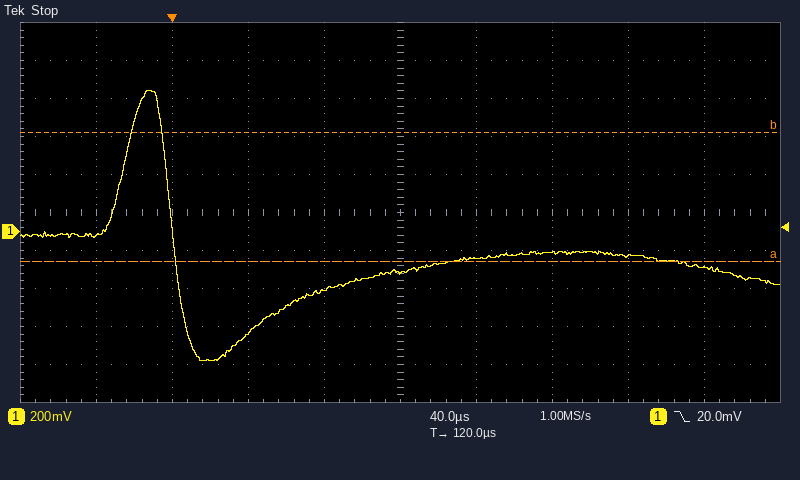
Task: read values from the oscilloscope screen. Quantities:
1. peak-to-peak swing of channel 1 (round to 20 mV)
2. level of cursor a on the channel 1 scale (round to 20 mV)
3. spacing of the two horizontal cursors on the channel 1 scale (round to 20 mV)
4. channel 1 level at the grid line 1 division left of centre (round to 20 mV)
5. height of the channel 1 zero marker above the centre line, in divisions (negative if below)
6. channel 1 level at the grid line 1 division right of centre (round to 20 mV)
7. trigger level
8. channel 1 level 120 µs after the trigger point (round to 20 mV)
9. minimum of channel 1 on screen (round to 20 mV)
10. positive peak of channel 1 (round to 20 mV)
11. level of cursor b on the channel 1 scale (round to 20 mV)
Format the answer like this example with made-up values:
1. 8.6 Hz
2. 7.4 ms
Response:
1. 1.42 V
2. -160 mV
3. 680 mV
4. -300 mV
5. -0.5 div
6. -140 mV
7. 20.0 mV
8. -220 mV
9. -680 mV
10. 740 mV
11. 520 mV
